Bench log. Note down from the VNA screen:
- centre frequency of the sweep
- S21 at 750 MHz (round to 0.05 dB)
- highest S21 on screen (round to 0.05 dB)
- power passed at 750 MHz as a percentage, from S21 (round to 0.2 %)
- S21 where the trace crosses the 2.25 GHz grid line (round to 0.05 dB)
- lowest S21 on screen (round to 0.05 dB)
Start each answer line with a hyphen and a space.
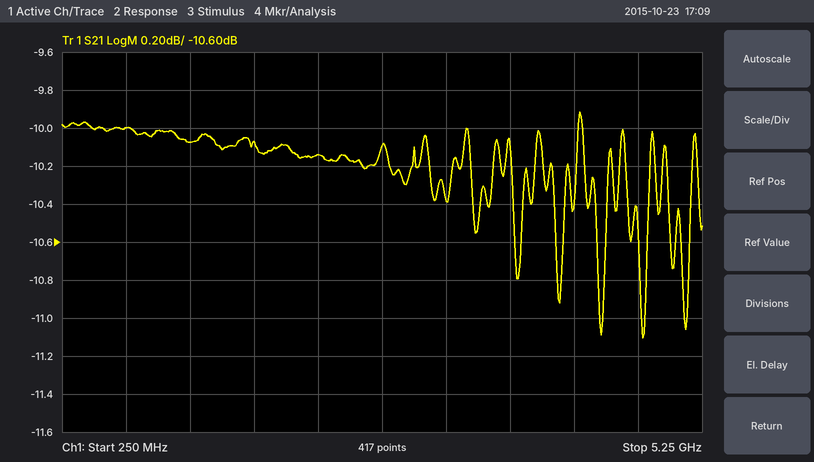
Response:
- 2.75 GHz
- -10.00 dB
- -9.90 dB
- 10.0 %
- -10.15 dB
- -11.10 dB
